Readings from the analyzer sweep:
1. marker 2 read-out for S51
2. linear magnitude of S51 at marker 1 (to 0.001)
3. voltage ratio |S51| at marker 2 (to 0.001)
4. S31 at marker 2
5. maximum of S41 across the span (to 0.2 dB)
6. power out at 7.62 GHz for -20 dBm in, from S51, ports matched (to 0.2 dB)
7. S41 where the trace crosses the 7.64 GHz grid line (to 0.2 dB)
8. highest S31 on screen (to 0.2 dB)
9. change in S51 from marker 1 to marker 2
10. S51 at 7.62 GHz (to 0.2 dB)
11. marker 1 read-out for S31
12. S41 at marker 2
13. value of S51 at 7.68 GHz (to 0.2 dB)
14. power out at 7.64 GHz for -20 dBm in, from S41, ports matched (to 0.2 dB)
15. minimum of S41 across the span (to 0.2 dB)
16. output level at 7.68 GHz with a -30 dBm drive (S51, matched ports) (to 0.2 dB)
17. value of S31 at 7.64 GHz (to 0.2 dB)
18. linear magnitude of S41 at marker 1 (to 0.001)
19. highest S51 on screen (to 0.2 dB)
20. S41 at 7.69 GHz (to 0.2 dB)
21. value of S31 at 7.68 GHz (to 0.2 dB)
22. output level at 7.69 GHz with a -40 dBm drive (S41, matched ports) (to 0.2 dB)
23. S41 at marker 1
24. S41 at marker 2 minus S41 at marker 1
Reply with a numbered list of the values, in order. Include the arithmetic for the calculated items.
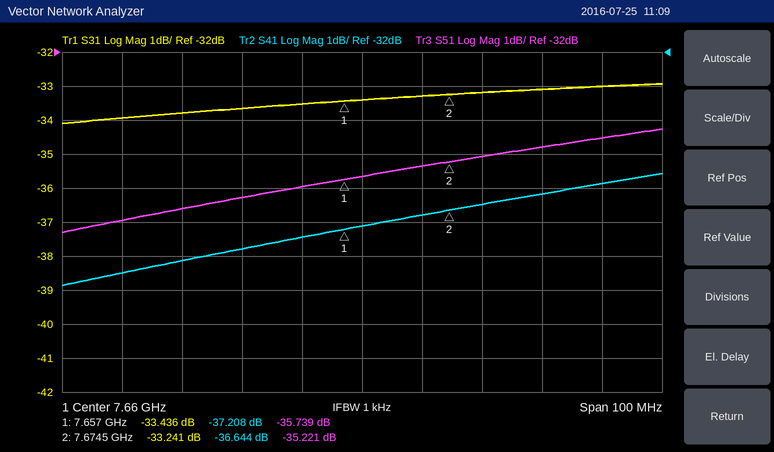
1. -35.221 dB
2. 10^(-35.739/20) ≈ 0.016
3. 10^(-35.221/20) ≈ 0.017
4. -33.241 dB
5. -35.6 dB
6. -20 dBm + (-37.0 dB) = -57.0 dBm
7. -37.8 dB
8. -33.0 dB
9. -35.221 − (-35.739) = 0.518 dB
10. -37.0 dB
11. -33.436 dB
12. -36.644 dB
13. -35.0 dB
14. -20 dBm + (-37.8 dB) = -57.8 dBm
15. -38.8 dB
16. -30 dBm + (-35.0 dB) = -65.0 dBm
17. -33.6 dB
18. 10^(-37.208/20) ≈ 0.014
19. -34.2 dB
20. -36.2 dB
21. -33.2 dB
22. -40 dBm + (-36.2 dB) = -76.2 dBm
23. -37.208 dB
24. -36.644 − (-37.208) = 0.564 dB
